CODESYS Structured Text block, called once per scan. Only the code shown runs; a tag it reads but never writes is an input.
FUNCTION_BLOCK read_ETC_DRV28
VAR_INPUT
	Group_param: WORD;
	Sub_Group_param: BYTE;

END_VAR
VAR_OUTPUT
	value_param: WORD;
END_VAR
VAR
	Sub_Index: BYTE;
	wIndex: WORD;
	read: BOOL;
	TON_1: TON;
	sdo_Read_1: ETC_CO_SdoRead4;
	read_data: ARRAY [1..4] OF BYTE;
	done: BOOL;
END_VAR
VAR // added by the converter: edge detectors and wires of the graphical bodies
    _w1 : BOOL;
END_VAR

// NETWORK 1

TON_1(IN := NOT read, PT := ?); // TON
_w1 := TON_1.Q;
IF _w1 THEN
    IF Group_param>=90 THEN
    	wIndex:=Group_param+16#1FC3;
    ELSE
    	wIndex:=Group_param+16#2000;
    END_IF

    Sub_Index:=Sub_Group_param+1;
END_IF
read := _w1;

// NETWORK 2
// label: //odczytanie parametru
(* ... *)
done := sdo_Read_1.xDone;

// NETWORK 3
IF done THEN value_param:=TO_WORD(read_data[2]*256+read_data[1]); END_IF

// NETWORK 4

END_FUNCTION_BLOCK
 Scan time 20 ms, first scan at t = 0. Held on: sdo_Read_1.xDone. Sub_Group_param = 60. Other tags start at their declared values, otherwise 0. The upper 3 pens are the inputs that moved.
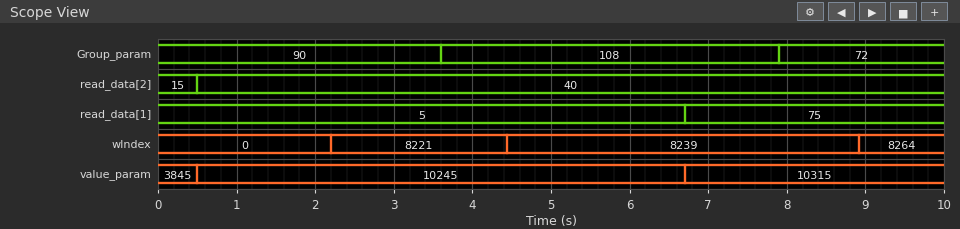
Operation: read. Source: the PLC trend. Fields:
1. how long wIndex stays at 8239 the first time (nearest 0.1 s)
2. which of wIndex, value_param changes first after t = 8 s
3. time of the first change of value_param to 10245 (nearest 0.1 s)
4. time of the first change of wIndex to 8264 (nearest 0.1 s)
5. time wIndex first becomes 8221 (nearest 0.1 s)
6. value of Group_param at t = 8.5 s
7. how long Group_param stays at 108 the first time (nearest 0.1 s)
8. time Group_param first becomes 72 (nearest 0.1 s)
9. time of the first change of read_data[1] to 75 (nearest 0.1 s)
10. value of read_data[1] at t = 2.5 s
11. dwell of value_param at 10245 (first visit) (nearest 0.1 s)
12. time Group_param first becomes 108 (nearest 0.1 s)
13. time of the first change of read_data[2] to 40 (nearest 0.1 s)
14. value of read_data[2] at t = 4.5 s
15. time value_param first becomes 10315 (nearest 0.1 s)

4.5 s
wIndex
0.5 s
8.9 s
2.2 s
72
4.3 s
7.9 s
6.7 s
5
6.2 s
3.6 s
0.5 s
40
6.7 s
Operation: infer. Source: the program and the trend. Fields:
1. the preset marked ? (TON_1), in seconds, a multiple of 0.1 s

2.2 s
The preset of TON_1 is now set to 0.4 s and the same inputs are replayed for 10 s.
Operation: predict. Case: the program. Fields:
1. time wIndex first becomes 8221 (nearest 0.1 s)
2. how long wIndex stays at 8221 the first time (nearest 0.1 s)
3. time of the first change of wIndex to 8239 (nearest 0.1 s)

0.4 s
3.5 s
3.9 s
